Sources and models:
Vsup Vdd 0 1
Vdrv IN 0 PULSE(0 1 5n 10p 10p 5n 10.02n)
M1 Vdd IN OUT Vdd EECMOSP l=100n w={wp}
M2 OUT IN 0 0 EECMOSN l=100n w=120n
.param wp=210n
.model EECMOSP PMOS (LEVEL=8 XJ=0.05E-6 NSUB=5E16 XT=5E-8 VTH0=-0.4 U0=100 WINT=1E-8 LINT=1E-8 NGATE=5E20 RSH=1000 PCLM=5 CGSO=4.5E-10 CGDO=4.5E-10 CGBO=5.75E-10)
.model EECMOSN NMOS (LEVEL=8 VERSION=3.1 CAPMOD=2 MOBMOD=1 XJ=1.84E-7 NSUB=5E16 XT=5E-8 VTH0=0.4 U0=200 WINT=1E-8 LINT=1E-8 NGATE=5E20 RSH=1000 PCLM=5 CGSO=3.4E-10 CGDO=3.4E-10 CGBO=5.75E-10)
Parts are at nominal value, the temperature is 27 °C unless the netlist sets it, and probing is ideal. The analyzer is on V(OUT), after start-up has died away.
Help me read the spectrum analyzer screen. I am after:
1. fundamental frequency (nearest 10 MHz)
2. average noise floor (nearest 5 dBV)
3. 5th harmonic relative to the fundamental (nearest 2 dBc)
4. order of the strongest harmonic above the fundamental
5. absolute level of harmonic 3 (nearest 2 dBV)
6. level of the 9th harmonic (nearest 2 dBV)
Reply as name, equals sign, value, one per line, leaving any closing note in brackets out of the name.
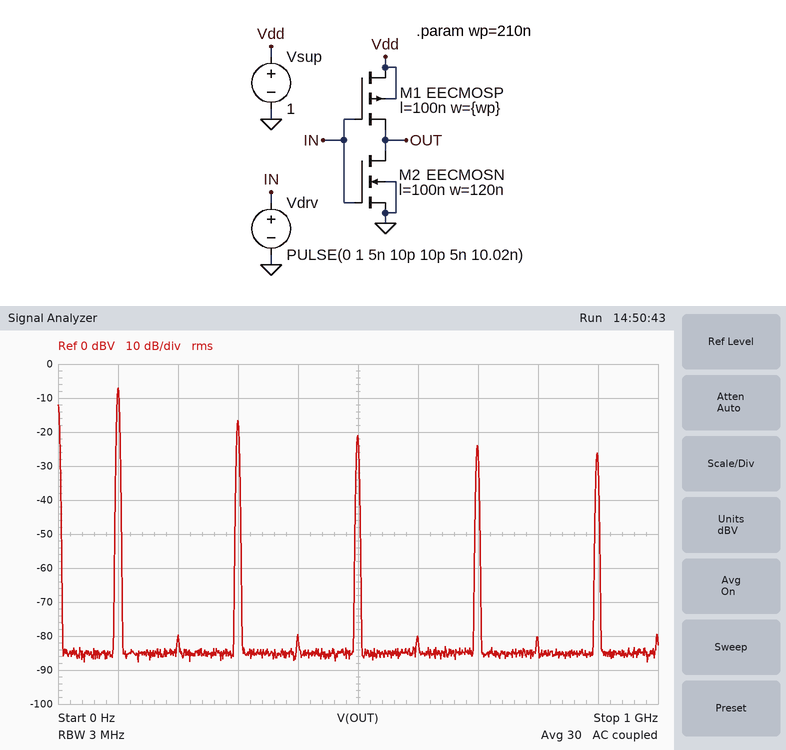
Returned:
fundamental frequency = 100 MHz
average noise floor = -85 dBV
5th harmonic relative to the fundamental = -14 dBc
order of the strongest harmonic above the fundamental = 3
absolute level of harmonic 3 = -16 dBV
level of the 9th harmonic = -26 dBV
